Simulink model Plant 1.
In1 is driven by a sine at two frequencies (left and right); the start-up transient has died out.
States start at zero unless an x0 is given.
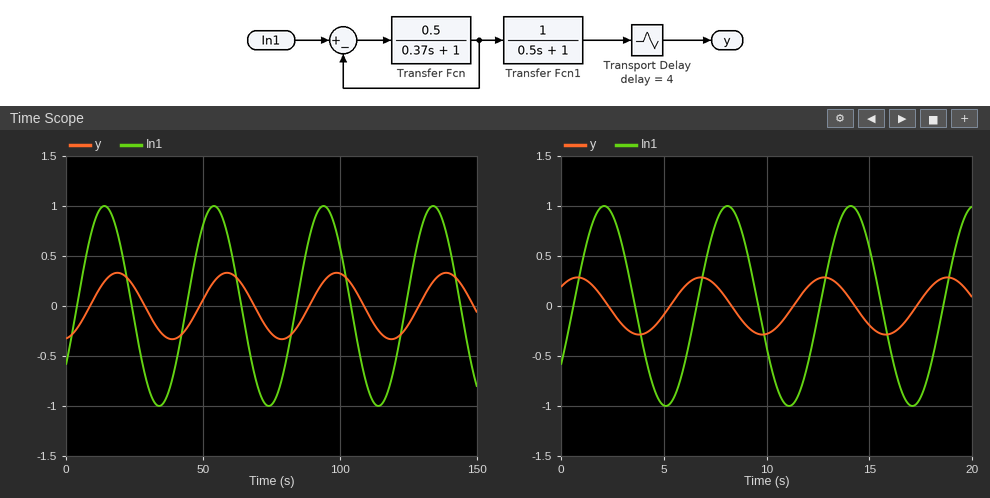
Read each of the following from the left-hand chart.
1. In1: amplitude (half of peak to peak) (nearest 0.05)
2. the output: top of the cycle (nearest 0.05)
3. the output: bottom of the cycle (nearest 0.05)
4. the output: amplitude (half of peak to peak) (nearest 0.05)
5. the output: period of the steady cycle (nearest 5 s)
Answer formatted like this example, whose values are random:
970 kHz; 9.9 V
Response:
1.00; 0.35; -0.35; 0.35; 40 s
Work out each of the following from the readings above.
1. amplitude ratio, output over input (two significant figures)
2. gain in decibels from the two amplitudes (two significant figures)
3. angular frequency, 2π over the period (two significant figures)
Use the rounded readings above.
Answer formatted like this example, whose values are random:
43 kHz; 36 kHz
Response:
0.35; -9.1 dB; 0.16 rad/s
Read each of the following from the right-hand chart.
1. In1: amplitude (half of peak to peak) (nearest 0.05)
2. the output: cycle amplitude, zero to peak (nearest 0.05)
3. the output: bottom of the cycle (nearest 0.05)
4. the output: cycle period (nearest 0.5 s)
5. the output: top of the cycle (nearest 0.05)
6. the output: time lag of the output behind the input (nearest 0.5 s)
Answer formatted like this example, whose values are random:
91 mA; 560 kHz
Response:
1.00; 0.30; -0.30; 6.0 s; 0.30; 4.5 s
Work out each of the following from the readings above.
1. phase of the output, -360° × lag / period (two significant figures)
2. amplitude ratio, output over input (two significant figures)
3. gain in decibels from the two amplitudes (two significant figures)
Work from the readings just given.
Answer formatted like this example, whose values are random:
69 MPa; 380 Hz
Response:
-270°; 0.30; -10 dB
